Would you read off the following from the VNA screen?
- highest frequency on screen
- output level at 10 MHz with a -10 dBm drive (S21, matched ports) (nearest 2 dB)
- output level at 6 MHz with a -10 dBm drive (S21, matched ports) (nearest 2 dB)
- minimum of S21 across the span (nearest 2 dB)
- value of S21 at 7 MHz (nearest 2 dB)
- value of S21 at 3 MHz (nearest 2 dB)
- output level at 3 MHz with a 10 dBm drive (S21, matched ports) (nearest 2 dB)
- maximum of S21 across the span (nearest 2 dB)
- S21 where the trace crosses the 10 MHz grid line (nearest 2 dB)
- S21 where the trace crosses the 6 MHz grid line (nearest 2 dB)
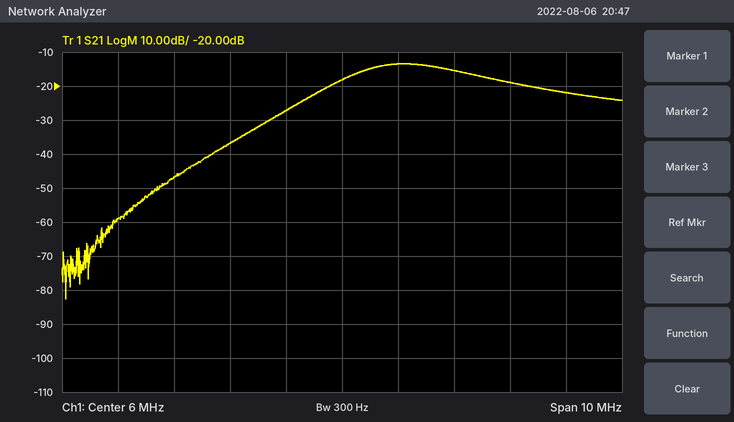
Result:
11 MHz
-32 dBm
-28 dBm
-82 dB
-14 dB
-46 dB
-36 dBm
-14 dB
-22 dB
-18 dB
